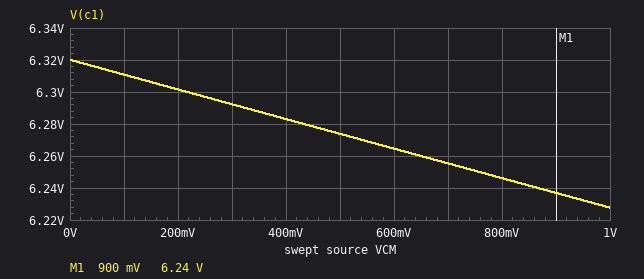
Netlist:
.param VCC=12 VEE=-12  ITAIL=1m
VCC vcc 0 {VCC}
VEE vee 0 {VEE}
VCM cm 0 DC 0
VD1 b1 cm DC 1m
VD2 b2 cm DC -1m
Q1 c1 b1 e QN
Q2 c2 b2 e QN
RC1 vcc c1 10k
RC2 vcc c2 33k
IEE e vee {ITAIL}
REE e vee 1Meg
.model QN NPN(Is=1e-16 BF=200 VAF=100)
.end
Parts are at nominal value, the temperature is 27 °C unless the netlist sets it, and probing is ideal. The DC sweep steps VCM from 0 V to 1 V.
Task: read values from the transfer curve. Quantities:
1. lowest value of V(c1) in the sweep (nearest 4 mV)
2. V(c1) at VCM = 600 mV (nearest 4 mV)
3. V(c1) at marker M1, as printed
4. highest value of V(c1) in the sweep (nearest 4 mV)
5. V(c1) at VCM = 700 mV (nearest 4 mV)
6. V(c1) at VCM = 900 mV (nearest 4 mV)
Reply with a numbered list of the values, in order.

1. 6.228 V
2. 6.264 V
3. 6.24 V
4. 6.320 V
5. 6.256 V
6. 6.236 V
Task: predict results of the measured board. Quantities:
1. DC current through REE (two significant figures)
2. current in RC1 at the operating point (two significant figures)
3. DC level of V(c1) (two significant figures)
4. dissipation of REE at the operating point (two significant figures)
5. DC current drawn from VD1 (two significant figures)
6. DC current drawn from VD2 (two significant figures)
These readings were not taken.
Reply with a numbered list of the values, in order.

1. 11 µA
2. 570 µA
3. 6.3 V
4. 130 µW
5. 2.7 µA
6. 56 µA
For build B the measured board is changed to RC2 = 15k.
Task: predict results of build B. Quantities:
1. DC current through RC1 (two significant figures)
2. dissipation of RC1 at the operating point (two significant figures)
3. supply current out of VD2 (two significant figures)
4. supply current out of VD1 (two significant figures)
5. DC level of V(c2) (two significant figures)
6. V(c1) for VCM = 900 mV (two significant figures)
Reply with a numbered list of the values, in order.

1. 530 µA
2. 2.8 mW
3. 2.3 µA
4. 2.5 µA
5. 4.8 V
6. 6.7 V
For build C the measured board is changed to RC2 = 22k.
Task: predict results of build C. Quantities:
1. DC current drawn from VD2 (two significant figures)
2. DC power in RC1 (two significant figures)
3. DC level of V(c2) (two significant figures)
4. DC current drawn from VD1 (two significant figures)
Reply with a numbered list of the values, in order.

1. 2.3 µA
2. 2.9 mW
3. 1.6 V
4. 2.5 µA
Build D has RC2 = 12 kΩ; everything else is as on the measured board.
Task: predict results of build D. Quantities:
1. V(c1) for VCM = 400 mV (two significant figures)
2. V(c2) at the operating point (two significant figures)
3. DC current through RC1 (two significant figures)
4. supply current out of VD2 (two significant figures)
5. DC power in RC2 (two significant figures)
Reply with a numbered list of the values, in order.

1. 6.8 V
2. 6.2 V
3. 520 µA
4. 2.3 µA
5. 2.8 mW
